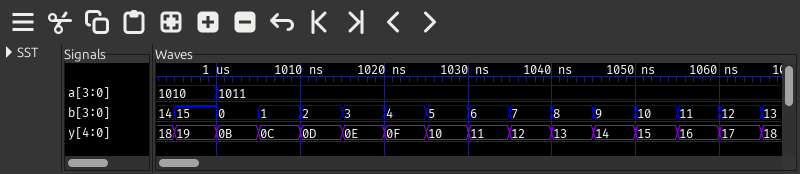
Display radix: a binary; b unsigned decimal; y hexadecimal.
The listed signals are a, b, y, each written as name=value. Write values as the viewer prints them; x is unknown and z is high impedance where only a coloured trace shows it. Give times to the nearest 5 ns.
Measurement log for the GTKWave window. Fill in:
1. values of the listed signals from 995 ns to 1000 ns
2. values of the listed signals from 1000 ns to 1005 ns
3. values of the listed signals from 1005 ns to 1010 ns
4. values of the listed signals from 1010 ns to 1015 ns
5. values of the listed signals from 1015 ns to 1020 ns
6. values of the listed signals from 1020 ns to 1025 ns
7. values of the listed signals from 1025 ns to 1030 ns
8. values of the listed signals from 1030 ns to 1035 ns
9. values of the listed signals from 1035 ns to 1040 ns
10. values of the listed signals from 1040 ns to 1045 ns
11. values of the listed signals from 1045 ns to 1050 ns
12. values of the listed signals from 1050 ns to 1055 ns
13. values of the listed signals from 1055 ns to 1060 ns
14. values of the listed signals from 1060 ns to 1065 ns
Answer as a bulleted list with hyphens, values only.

- a=1010, b=15, y=19
- a=1011, b=0, y=0B
- a=1011, b=1, y=0C
- a=1011, b=2, y=0D
- a=1011, b=3, y=0E
- a=1011, b=4, y=0F
- a=1011, b=5, y=10
- a=1011, b=6, y=11
- a=1011, b=7, y=12
- a=1011, b=8, y=13
- a=1011, b=9, y=14
- a=1011, b=10, y=15
- a=1011, b=11, y=16
- a=1011, b=12, y=17
